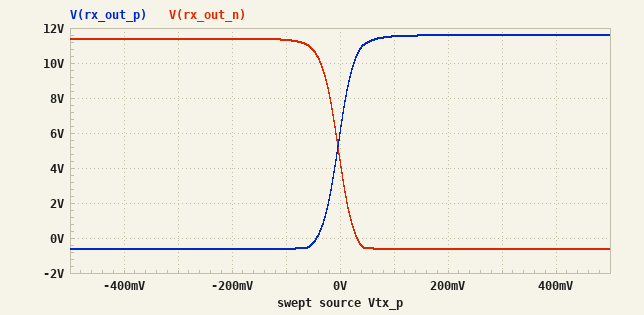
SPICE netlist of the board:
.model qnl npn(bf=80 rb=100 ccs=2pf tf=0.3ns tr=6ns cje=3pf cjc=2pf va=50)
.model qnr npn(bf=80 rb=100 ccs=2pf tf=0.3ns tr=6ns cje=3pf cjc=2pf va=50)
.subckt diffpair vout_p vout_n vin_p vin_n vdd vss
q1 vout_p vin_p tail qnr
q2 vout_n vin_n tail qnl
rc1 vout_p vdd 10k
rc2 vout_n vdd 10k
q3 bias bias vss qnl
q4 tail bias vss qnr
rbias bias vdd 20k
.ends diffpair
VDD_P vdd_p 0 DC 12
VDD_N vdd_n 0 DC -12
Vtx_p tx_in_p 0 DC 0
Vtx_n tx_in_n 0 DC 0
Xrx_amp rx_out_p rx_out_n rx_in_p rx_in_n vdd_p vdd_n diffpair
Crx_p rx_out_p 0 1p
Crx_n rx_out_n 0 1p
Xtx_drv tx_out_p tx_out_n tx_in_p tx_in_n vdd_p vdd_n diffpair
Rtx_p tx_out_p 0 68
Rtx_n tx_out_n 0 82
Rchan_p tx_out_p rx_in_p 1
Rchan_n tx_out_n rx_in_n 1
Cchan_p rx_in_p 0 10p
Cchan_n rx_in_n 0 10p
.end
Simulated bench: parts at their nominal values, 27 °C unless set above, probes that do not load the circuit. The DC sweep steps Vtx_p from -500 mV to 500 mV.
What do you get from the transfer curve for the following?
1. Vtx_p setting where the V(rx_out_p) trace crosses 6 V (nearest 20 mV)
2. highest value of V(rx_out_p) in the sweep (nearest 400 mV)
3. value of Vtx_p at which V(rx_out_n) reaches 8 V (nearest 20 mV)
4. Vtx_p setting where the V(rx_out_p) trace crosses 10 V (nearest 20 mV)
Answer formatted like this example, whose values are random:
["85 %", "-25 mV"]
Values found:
["0 V", "11.6 V", "-20 mV", "20 mV"]
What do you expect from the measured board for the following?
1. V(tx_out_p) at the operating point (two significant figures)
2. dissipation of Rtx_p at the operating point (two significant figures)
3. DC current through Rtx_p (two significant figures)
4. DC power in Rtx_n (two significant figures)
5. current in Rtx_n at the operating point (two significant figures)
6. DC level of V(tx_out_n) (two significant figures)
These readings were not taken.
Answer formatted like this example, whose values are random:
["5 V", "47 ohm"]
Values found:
["35 mV", "18 µW", "510 µA", "21 µW", "510 µA", "42 mV"]
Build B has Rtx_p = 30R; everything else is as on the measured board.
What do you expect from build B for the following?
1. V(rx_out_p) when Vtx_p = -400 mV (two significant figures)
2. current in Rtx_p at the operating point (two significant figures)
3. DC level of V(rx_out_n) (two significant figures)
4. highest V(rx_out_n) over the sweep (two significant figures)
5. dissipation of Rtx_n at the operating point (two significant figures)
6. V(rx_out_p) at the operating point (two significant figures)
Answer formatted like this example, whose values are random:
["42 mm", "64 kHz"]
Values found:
["650 mV", "520 µA", "2.4 V", "9.8 V", "21 µW", "8.0 V"]
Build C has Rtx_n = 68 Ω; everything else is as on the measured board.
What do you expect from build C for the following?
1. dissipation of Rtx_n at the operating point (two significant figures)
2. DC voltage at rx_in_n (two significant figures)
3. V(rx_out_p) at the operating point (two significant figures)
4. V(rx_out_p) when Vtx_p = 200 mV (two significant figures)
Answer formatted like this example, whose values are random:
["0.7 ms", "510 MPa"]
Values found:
["18 µW", "35 mV", "5.2 V", "11 V"]
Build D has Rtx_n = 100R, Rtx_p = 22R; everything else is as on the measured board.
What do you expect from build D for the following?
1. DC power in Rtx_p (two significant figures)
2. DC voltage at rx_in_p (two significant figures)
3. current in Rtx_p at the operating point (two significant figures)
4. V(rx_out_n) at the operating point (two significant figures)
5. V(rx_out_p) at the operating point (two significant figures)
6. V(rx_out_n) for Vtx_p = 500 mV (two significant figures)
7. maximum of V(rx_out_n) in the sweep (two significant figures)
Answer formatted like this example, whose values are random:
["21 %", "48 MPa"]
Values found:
["5.9 µW", "11 mV", "520 µA", "1.3 V", "9.2 V", "-600 mV", "9.3 V"]
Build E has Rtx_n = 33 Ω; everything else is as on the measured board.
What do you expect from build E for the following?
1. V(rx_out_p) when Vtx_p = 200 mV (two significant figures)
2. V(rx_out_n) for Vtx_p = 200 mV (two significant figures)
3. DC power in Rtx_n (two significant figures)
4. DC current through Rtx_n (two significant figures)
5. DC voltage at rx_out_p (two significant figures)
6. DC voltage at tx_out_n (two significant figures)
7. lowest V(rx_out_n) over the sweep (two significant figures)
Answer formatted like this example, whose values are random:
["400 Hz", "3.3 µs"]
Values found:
["9.9 V", "550 mV", "8.8 µW", "520 µA", "3.3 V", "17 mV", "520 mV"]
